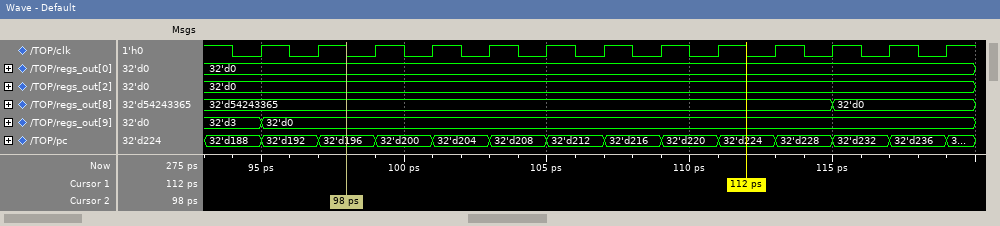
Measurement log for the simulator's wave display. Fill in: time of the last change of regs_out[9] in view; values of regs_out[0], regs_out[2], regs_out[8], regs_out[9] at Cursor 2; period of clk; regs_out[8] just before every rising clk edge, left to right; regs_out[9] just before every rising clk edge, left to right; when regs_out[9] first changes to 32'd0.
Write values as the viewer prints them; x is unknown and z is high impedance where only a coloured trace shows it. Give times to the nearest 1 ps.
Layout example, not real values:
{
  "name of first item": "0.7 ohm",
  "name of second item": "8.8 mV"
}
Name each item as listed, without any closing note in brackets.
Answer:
{
  "time of the last change of regs_out[9] in view": "95 ps",
  "values of regs_out[0], regs_out[2], regs_out[8], regs_out[9] at Cursor 2": "regs_out[0]=32'd0, regs_out[2]=32'd0, regs_out[8]=32'd54243365, regs_out[9]=32'd0",
  "period of clk": "2 ps",
  "regs_out[8] just before every rising clk edge, left to right": "32'd54243365, 32'd54243365, 32'd54243365, 32'd54243365, 32'd54243365, 32'd54243365, 32'd54243365, 32'd54243365, 32'd54243365, 32'd54243365, 32'd54243365, 32'd0, 32'd0",
  "regs_out[9] just before every rising clk edge, left to right": "32'd3, 32'd0, 32'd0, 32'd0, 32'd0, 32'd0, 32'd0, 32'd0, 32'd0, 32'd0, 32'd0, 32'd0, 32'd0",
  "when regs_out[9] first changes to 32'd0": "95 ps"
}
